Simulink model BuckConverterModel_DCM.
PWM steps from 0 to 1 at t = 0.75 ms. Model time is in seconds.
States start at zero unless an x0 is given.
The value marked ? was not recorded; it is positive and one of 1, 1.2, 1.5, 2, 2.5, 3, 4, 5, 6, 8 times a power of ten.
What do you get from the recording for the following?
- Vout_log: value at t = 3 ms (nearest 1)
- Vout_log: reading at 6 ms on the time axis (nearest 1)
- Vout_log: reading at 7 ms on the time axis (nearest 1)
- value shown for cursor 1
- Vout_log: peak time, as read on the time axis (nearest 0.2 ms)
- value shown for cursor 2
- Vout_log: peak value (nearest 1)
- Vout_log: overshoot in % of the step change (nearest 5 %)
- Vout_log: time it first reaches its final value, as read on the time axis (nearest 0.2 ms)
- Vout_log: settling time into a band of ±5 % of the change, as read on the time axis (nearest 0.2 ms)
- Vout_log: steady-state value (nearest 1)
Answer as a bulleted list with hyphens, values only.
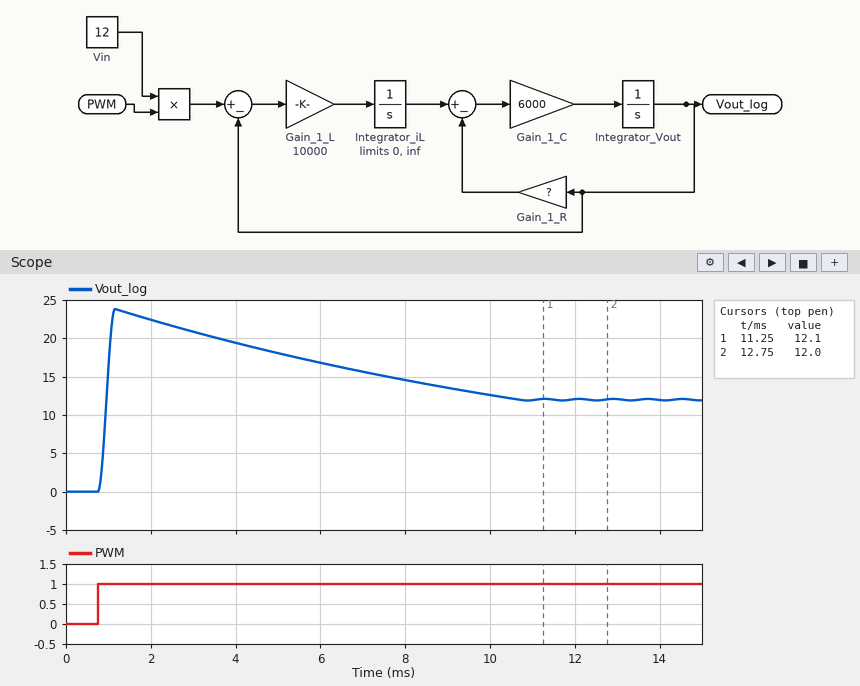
- 21
- 17
- 16
- 12.1
- 1.2 ms
- 12.0
- 24
- 100 %
- 1.0 ms
- 10.0 ms
- 12
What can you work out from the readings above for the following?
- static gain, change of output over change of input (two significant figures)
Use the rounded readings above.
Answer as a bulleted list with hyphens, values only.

- 12
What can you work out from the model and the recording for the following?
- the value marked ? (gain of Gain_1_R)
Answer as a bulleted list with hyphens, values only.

- 0.012
